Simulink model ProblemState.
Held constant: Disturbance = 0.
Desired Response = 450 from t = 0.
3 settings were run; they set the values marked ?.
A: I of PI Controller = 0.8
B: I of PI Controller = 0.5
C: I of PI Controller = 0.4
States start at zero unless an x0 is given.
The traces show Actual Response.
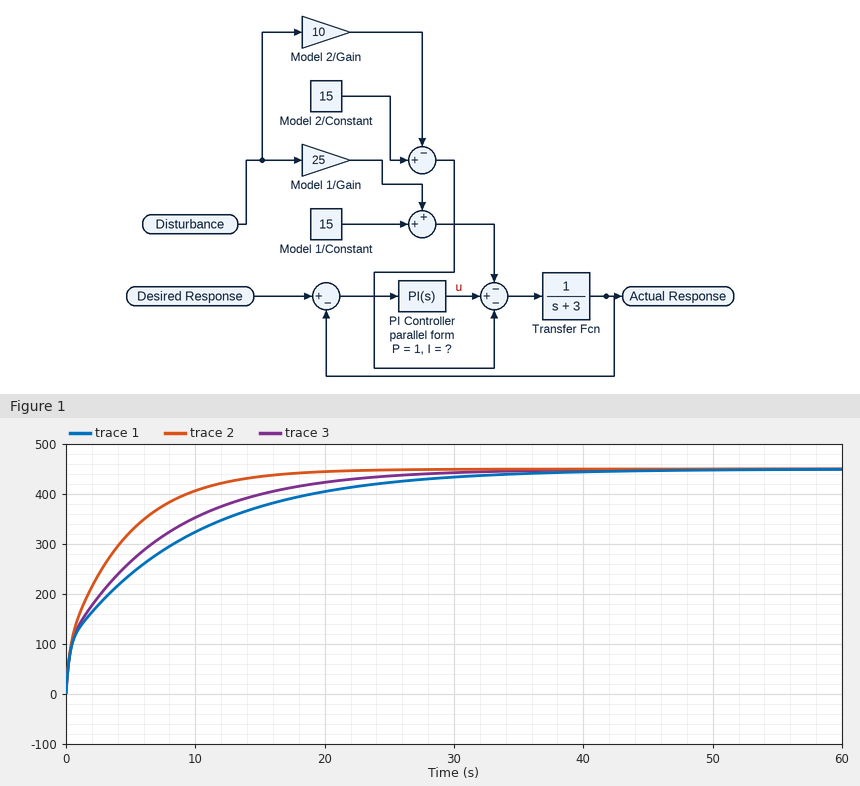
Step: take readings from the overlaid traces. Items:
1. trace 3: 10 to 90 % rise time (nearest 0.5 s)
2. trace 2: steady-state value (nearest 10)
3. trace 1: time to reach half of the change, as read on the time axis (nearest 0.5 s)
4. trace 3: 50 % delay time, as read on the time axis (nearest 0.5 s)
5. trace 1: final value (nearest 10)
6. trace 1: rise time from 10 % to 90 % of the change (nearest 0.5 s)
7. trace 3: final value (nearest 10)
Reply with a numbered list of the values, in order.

1. 16.0 s
2. 450
3. 4.5 s
4. 3.5 s
5. 450
6. 20.0 s
7. 450
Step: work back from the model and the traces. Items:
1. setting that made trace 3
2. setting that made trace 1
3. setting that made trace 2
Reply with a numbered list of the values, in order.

1. B
2. C
3. A
